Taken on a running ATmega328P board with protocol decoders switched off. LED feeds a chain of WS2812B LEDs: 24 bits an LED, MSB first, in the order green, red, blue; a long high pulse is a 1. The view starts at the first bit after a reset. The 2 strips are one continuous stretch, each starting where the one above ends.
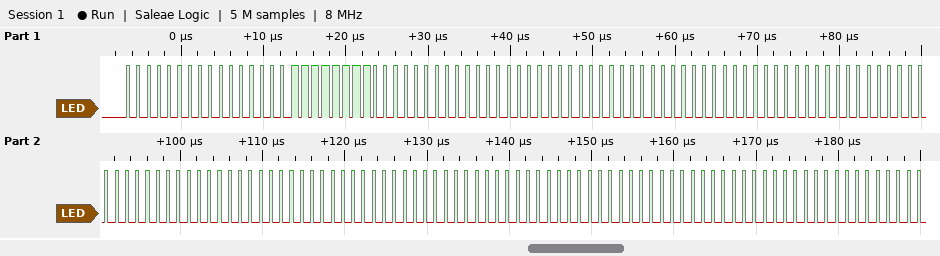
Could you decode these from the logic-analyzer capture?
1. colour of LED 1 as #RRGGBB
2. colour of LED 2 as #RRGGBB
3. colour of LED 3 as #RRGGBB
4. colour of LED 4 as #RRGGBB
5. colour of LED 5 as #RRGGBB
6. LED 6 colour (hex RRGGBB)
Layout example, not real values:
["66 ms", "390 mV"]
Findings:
["#0000FF", "#000000", "#000000", "#000000", "#000000", "#000000"]
